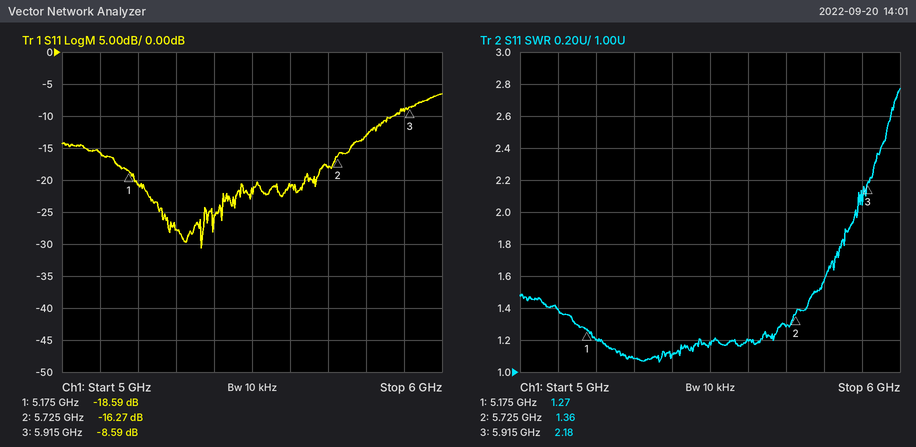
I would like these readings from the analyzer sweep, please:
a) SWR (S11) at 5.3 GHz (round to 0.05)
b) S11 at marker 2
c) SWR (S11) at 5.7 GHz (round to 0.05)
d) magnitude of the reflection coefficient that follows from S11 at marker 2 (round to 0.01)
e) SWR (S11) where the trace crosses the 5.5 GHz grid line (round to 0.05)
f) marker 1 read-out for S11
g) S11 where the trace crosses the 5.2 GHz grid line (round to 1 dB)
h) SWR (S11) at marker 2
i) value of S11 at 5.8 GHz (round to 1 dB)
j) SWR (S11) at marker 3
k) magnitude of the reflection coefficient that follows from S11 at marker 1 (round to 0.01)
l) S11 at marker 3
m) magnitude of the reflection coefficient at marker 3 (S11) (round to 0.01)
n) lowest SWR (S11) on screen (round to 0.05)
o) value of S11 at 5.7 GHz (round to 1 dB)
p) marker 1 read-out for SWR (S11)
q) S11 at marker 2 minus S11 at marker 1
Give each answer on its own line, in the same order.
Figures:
1.10
-16.27 dB
1.30
0.15
1.20
-18.59 dB
-21 dB
1.36
-13 dB
2.18
0.12
-8.59 dB
0.37
1.05
-18 dB
1.27
2.32 dB
